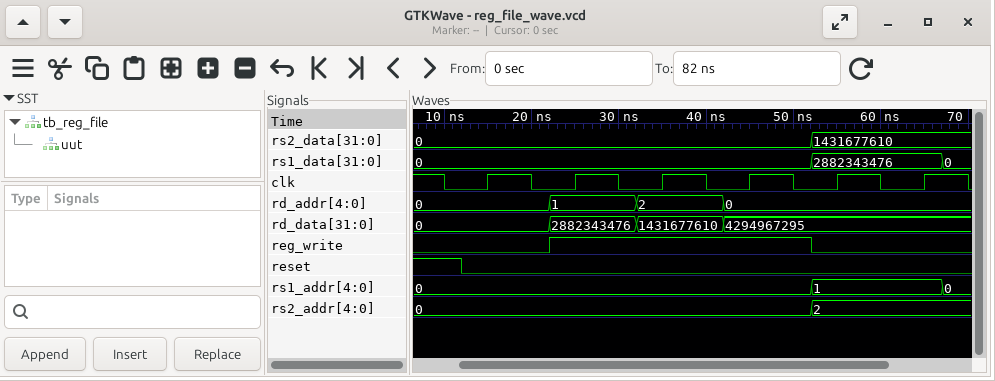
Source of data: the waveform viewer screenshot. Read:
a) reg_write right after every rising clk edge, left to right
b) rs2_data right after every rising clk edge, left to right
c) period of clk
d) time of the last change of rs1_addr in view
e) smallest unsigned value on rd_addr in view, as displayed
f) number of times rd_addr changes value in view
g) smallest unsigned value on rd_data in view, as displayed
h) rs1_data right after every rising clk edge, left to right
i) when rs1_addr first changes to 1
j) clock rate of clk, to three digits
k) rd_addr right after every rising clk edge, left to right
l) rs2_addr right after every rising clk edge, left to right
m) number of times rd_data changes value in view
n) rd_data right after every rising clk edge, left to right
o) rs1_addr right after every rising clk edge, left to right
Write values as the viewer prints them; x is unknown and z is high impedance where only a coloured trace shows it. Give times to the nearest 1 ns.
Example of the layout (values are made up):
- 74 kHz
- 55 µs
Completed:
- 0 1 1 1 0 0
- 0, 0, 0, 0, 1431677610, 1431677610
- 10 ns
- 67 ns
- 0
- 3
- 0
- 0, 0, 0, 0, 2882343476, 2882343476
- 52 ns
- 100 MHz
- 0, 1, 2, 0, 0, 0
- 0, 0, 0, 0, 2, 2
- 3
- 0, 2882343476, 1431677610, 4294967295, 4294967295, 4294967295
- 0, 0, 0, 0, 1, 1
